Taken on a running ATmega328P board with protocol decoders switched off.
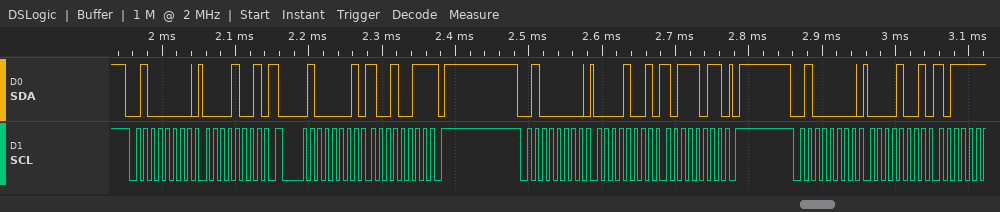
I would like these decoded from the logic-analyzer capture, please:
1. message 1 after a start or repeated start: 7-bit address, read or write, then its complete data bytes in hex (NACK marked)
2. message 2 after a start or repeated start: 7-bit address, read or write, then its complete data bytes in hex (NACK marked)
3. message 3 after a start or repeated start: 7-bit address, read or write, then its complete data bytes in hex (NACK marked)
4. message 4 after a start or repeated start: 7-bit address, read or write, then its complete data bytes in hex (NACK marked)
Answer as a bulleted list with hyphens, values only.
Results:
- 0x20 write: 09
- 0x20 read: 93 NACK
- 0x20 write: 09 BB
- 0x20 write: 09
